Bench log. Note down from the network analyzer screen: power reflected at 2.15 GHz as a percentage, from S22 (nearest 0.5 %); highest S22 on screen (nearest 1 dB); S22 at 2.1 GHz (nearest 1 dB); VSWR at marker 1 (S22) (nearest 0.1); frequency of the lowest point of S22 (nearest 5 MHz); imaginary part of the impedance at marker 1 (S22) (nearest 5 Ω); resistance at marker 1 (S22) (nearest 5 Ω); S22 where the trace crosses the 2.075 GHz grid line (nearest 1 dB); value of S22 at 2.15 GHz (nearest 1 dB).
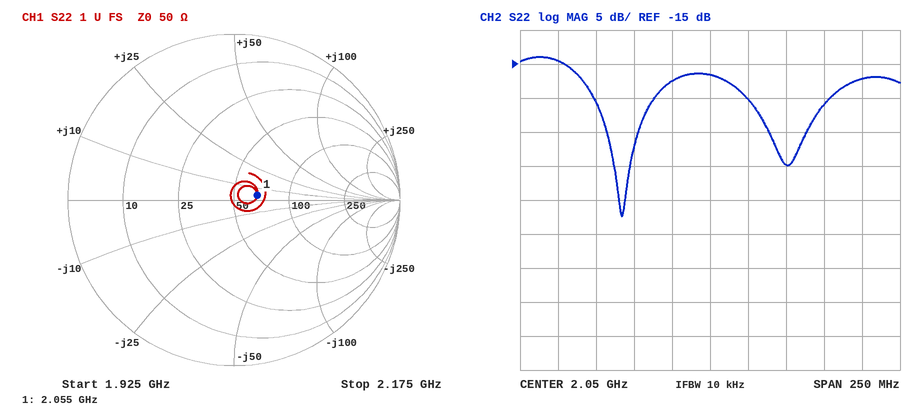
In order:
2.0 %
-14 dB
-30 dB
1.3
1.990 GHz
+5 Ω
65 Ω
-20 dB
-17 dB
